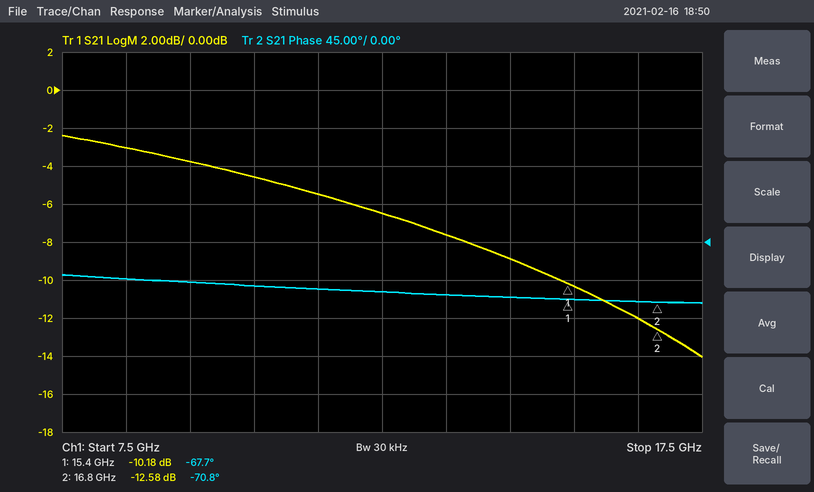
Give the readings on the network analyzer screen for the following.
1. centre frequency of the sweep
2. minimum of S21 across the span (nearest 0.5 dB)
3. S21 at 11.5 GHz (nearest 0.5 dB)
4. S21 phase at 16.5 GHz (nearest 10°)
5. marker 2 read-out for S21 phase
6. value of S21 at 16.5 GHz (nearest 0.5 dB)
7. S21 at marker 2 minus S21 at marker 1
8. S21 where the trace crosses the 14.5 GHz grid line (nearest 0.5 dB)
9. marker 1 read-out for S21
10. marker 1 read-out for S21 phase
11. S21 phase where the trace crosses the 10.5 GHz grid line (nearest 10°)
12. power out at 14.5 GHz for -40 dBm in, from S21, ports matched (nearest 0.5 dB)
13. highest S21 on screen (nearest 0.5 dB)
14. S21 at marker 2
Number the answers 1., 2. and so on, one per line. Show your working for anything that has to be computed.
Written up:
1. 12.5 GHz
2. -14.0 dB
3. -5.5 dB
4. -70°
5. -70.8°
6. -12.0 dB
7. -12.58 − (-10.18) = -2.40 dB
8. -9.0 dB
9. -10.18 dB
10. -67.7°
11. -50°
12. -40 dBm + (-9.0 dB) = -49.0 dBm
13. -2.5 dB
14. -12.58 dB
